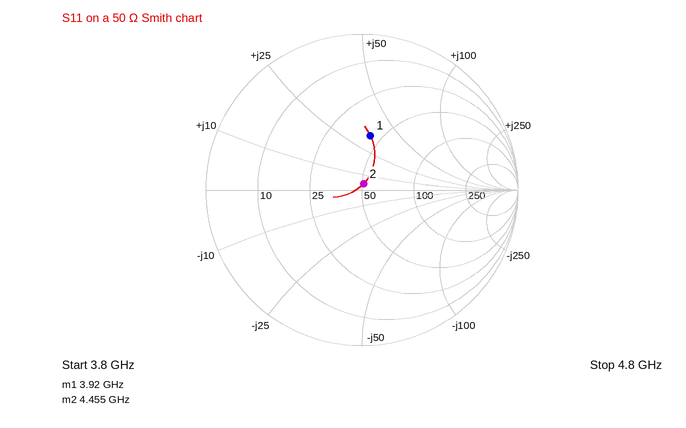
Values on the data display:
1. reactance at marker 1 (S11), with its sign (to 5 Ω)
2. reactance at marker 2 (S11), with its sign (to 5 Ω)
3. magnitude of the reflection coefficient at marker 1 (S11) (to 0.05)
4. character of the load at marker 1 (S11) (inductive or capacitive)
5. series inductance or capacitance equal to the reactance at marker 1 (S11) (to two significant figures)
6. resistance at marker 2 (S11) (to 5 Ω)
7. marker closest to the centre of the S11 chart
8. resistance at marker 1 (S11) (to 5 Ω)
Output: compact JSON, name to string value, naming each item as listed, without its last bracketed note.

{"reactance at marker 1 (S11), with its sign": "+35 Ω", "reactance at marker 2 (S11), with its sign": "+5 Ω", "magnitude of the reflection coefficient at marker 1 (S11)": "0.35", "character of the load at marker 1 (S11)": "inductive", "series inductance or capacitance equal to the reactance at marker 1 (S11)": "1.4 nH", "resistance at marker 2 (S11)": "50 Ω", "marker closest to the centre of the S11 chart": "marker 2", "resistance at marker 1 (S11)": "45 Ω"}
